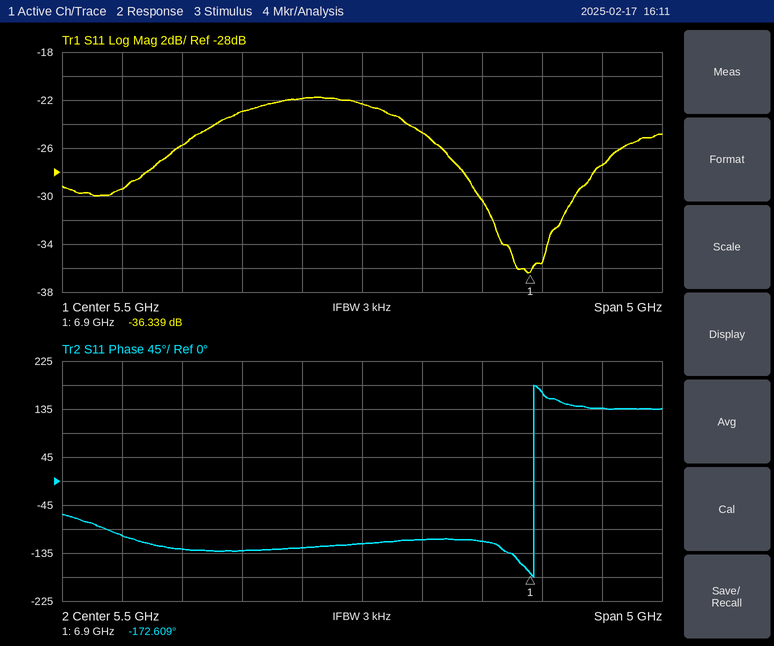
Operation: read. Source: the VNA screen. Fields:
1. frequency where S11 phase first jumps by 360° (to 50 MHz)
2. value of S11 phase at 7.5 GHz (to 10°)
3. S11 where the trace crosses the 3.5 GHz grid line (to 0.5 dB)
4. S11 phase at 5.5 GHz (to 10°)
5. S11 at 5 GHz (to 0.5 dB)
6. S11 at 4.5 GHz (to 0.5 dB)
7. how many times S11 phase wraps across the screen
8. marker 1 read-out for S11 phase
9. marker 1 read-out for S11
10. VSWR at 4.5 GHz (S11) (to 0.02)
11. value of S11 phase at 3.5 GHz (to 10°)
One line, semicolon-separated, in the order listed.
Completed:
6.95 GHz; 140°; -29.5 dB; -120°; -22.0 dB; -23.0 dB; 1; -172.609°; -36.339 dB; 1.16; -100°
